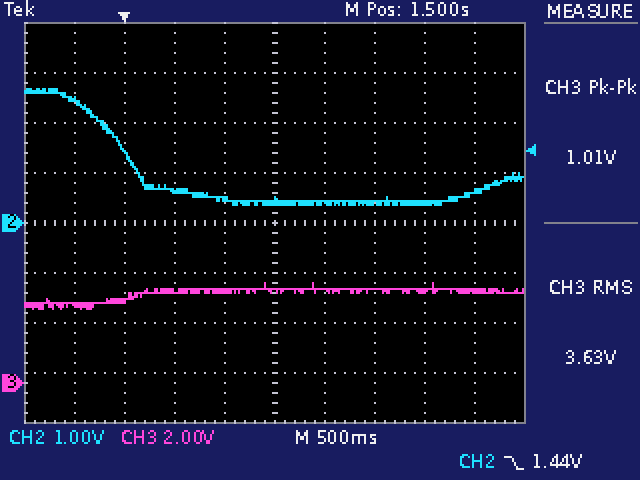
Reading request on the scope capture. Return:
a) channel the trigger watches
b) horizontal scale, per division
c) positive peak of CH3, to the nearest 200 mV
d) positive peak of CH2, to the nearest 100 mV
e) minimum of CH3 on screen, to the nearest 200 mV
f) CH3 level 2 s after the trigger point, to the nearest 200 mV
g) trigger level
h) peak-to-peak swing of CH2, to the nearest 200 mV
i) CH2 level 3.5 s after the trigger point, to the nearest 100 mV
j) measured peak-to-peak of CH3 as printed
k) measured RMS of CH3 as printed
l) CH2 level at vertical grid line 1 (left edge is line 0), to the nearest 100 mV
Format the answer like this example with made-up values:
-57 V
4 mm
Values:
CH2
500 ms
4.0 V
2.7 V
3.0 V
3.8 V
1.44 V
2.4 V
600 mV
1.01 V
3.63 V
2.4 V
